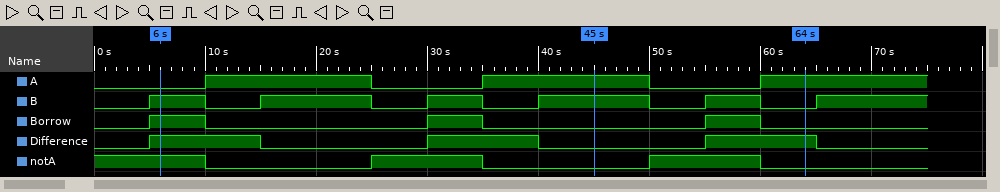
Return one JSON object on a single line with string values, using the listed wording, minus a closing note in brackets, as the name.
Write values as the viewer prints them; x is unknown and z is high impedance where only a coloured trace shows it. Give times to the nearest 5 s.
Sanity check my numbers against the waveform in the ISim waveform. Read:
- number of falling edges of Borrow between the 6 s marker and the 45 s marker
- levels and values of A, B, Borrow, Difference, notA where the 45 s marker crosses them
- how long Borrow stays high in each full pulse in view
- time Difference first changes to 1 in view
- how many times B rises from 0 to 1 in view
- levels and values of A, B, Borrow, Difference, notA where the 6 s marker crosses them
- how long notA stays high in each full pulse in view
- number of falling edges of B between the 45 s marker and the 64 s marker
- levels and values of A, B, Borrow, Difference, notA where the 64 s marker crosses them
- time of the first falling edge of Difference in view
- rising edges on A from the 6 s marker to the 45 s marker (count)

{"number of falling edges of Borrow between the 6 s marker and the 45 s marker": "2", "levels and values of A, B, Borrow, Difference, notA where the 45 s marker crosses them": "A=1, B=1, Borrow=0, Difference=0, notA=0", "how long Borrow stays high in each full pulse in view": "5 s, 5 s, 5 s", "time Difference first changes to 1 in view": "5 s", "how many times B rises from 0 to 1 in view": "6", "levels and values of A, B, Borrow, Difference, notA where the 6 s marker crosses them": "A=0, B=1, Borrow=1, Difference=1, notA=1", "how long notA stays high in each full pulse in view": "10 s, 10 s", "number of falling edges of B between the 45 s marker and the 64 s marker": "2", "levels and values of A, B, Borrow, Difference, notA where the 64 s marker crosses them": "A=1, B=0, Borrow=0, Difference=1, notA=0", "time of the first falling edge of Difference in view": "15 s", "rising edges on A from the 6 s marker to the 45 s marker": "2"}
